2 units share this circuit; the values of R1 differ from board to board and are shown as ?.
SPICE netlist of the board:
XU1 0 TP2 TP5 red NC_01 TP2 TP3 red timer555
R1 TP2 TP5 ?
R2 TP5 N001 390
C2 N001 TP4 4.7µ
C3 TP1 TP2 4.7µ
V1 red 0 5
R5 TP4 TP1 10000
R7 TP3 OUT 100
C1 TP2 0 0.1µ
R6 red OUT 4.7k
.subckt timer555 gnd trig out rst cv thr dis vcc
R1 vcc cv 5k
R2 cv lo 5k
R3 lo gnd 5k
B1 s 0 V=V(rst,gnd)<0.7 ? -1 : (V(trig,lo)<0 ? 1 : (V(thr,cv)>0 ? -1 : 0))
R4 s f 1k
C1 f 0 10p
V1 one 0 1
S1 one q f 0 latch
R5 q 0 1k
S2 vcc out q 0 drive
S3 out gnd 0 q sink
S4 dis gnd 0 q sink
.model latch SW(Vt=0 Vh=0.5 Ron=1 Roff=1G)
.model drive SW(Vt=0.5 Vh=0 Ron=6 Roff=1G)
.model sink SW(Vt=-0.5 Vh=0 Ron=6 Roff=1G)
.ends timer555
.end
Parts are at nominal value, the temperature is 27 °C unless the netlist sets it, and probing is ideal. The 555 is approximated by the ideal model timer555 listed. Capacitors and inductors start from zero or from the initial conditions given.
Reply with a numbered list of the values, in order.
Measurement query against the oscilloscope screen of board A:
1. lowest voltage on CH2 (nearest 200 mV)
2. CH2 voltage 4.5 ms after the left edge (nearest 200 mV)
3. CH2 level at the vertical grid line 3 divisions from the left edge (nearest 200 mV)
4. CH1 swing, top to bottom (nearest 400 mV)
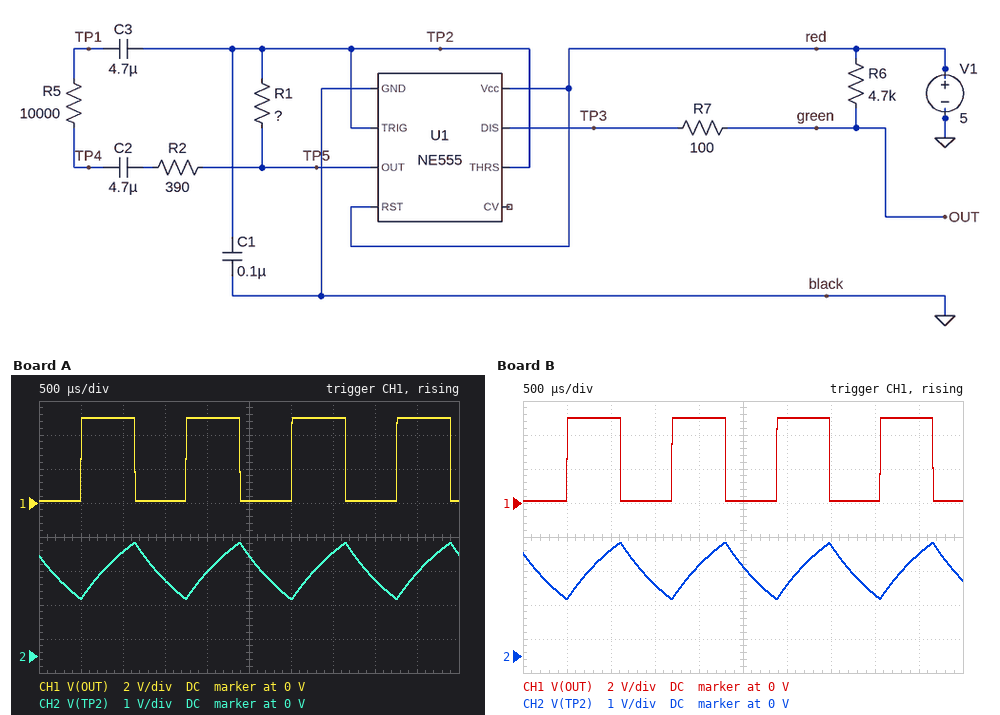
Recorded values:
1. 1.6 V
2. 2.4 V
3. 2.2 V
4. 4.8 V
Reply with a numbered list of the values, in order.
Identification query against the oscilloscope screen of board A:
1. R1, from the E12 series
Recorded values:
1. 68 kΩ
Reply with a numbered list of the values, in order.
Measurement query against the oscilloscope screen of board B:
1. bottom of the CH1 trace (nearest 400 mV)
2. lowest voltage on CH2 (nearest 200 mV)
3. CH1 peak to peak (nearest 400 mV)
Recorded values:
1. 0 V
2. 1.6 V
3. 4.8 V
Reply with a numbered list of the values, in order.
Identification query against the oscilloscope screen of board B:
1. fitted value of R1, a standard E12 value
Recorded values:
1. 47 kΩ
